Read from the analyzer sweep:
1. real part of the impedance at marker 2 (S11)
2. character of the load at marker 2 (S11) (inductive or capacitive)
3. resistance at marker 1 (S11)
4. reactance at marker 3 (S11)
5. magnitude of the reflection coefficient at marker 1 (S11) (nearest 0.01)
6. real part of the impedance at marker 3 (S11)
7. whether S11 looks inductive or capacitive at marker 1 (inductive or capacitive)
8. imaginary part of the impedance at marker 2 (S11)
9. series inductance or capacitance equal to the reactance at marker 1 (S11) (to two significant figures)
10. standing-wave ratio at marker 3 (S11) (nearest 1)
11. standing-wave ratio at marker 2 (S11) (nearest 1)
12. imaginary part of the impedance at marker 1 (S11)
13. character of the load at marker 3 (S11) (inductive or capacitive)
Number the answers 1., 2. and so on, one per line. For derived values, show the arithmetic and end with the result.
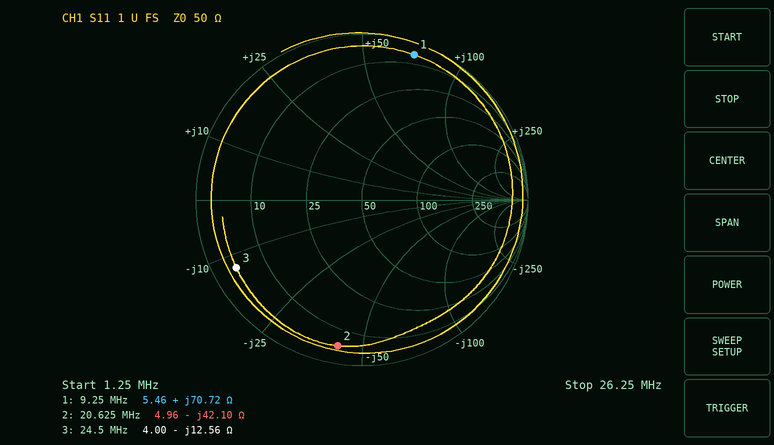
1. 4.96 Ω
2. capacitive
3. 5.46 Ω
4. -12.56 Ω
5. 0.93
6. 4.00 Ω
7. inductive
8. -42.10 Ω
9. L = 70.72 Ω/(2π × 9.25 MHz) ≈ 1.2 µH
10. 13
11. 17
12. +70.72 Ω
13. capacitive
